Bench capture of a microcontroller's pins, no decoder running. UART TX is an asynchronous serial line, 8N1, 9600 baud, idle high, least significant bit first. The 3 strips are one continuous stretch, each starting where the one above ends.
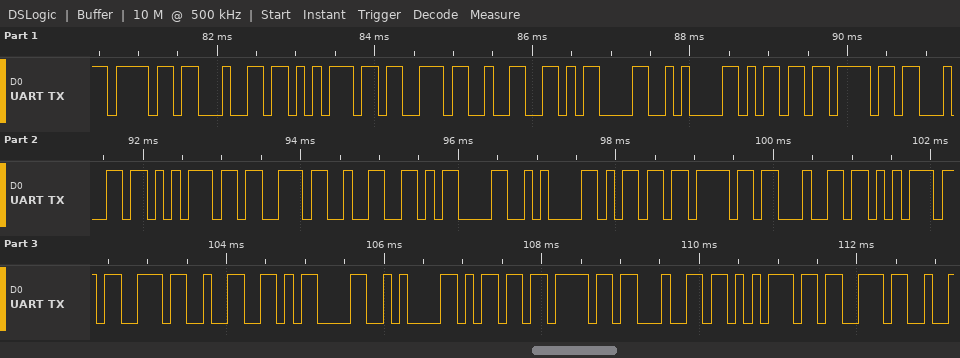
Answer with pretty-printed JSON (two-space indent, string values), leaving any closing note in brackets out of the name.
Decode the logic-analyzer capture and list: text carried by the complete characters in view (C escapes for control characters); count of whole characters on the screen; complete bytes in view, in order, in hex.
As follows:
{
  "text carried by the complete characters in view": "\"odus2\\r\\nmodus2\\r\\nmodus2\\r\\nmodus\"",
  "count of whole characters on the screen": "28",
  "complete bytes in view, in order, in hex": "0x6F 0x64 0x75 0x73 0x32 0x0D 0x0A 0x6D 0x6F 0x64 0x75 0x73 0x32 0x0D 0x0A 0x6D 0x6F 0x64 0x75 0x73 0x32 0x0D 0x0A 0x6D 0x6F 0x64 0x75 0x73"
}
